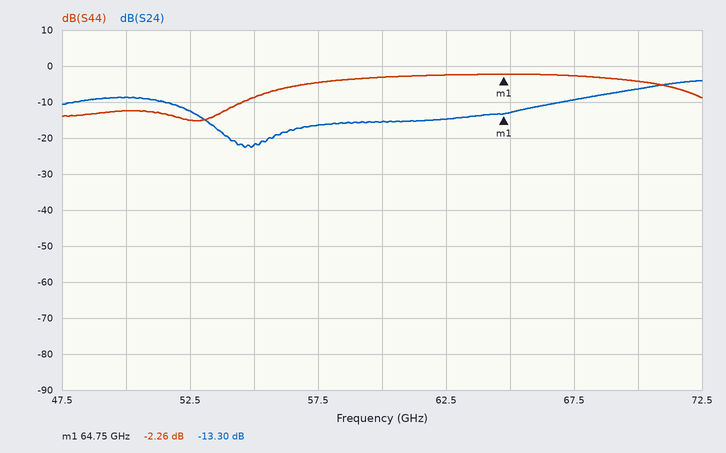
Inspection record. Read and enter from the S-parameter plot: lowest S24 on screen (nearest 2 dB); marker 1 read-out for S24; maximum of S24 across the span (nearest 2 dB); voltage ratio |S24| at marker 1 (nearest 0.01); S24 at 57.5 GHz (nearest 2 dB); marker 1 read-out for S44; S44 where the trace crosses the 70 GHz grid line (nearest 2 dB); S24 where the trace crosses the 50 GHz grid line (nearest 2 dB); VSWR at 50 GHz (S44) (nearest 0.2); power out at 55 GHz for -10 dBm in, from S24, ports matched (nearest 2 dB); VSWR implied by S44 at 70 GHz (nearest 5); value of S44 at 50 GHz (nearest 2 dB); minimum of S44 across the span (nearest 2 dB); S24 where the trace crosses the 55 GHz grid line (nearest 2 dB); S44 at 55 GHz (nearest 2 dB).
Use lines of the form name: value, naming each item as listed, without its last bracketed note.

lowest S24 on screen: -22 dB
marker 1 read-out for S24: -13.30 dB
maximum of S24 across the span: -4 dB
voltage ratio |S24| at marker 1: 0.22
S24 at 57.5 GHz: -16 dB
marker 1 read-out for S44: -2.26 dB
S44 where the trace crosses the 70 GHz grid line: -4 dB
S24 where the trace crosses the 50 GHz grid line: -8 dB
VSWR at 50 GHz (S44): 1.6
power out at 55 GHz for -10 dBm in, from S24, ports matched: -32 dBm
VSWR implied by S44 at 70 GHz: 5
value of S44 at 50 GHz: -12 dB
minimum of S44 across the span: -16 dB
S24 where the trace crosses the 55 GHz grid line: -22 dB
S44 at 55 GHz: -8 dB
